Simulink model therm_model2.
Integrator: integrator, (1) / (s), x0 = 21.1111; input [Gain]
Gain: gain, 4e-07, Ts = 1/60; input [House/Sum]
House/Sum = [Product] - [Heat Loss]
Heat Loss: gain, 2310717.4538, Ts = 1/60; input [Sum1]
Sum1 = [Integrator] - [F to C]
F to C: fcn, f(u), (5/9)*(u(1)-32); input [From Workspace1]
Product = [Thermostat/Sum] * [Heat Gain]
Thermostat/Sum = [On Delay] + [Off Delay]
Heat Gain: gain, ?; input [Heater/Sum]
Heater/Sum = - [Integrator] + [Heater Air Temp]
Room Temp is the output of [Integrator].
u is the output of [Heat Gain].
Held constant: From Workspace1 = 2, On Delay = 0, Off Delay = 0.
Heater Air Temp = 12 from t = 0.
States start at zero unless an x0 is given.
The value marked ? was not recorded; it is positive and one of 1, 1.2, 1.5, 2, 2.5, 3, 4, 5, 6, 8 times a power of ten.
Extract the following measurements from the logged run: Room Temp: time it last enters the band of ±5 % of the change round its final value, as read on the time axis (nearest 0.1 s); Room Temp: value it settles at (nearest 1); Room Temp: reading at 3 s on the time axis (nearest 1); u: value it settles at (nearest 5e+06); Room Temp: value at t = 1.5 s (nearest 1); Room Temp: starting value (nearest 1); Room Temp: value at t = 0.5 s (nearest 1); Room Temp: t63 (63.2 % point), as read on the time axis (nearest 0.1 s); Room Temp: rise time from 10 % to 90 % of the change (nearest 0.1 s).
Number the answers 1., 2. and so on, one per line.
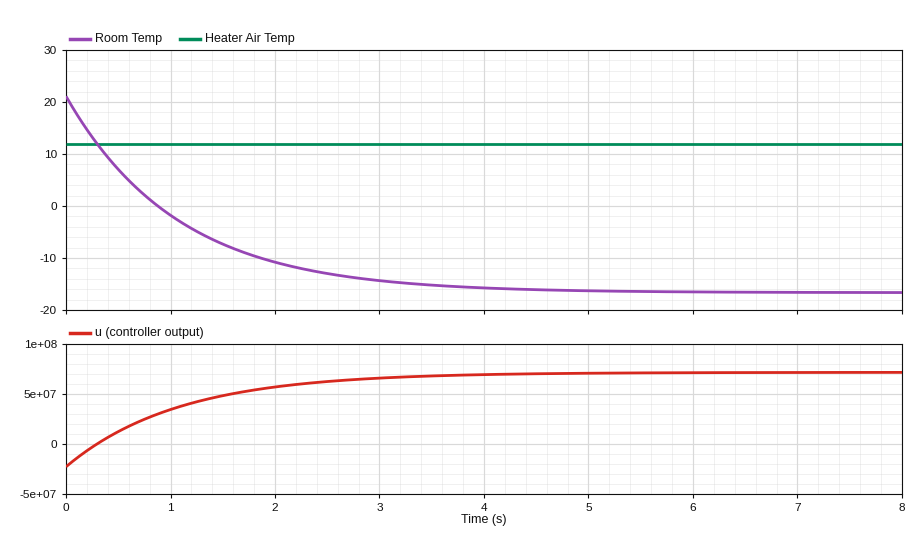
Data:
1. 3.2 s
2. -17
3. -14
4. 70000000
5. -7
6. 21
7. 7
8. 1.1 s
9. 2.4 s
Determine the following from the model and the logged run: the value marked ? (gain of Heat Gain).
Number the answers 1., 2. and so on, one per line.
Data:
1. 2.5e+06
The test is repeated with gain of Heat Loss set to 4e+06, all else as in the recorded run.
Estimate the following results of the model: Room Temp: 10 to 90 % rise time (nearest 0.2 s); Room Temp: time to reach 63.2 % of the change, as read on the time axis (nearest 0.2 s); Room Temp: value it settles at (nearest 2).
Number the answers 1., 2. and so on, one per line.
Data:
1. 1.4 s
2. 0.6 s
3. -16
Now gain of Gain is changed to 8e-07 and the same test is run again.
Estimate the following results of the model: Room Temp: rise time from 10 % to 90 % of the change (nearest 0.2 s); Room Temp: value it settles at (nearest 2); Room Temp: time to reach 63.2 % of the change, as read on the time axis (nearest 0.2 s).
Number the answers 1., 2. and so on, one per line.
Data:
1. 1.2 s
2. -16
3. 0.6 s
